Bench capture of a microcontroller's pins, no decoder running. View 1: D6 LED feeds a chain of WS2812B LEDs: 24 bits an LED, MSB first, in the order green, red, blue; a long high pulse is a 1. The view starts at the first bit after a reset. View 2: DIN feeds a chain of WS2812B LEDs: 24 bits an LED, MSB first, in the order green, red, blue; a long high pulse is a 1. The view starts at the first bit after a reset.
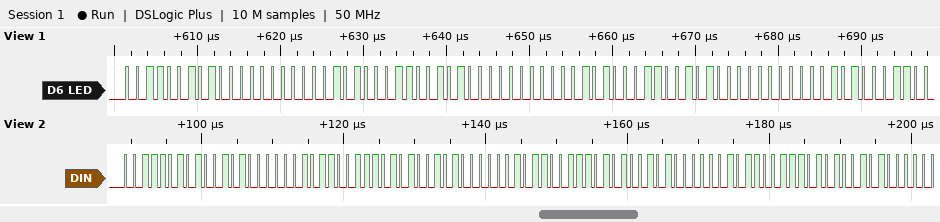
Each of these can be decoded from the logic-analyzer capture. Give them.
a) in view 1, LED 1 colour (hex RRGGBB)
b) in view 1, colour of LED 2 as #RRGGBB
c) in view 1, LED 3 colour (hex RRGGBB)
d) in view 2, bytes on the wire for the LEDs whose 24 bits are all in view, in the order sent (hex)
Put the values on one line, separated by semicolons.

#80320A; #80320A; #80320A; 3A 94 0B 3A 94 0B 3A 94 0B
